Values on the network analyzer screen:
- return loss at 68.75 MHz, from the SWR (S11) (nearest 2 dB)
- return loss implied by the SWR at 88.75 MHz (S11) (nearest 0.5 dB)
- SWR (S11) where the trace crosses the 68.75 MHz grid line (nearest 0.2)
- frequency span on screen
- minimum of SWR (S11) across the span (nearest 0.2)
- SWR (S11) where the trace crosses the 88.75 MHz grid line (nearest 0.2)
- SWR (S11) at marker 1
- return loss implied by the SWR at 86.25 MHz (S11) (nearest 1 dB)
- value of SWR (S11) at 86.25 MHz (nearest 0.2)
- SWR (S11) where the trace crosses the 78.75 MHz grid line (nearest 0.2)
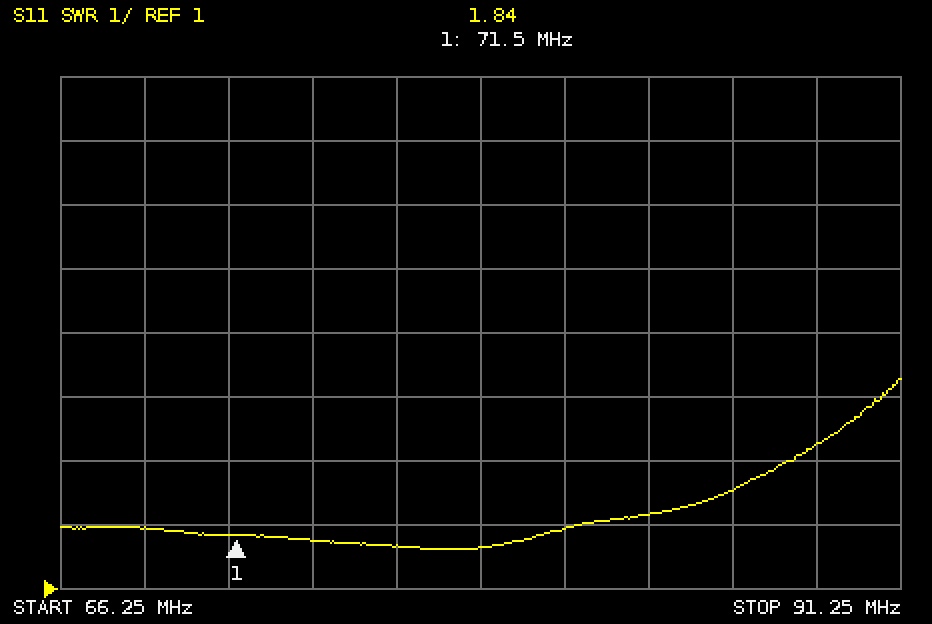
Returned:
10 dB
5.5 dB
2.0
25 MHz
1.6
3.2
1.84
7 dB
2.6
1.6
